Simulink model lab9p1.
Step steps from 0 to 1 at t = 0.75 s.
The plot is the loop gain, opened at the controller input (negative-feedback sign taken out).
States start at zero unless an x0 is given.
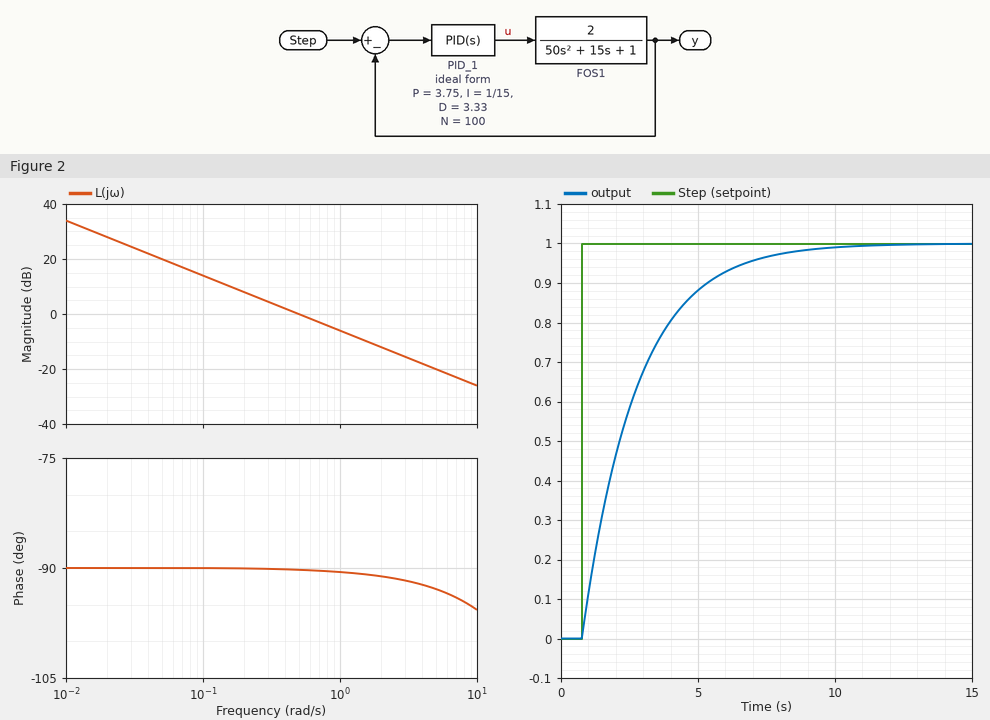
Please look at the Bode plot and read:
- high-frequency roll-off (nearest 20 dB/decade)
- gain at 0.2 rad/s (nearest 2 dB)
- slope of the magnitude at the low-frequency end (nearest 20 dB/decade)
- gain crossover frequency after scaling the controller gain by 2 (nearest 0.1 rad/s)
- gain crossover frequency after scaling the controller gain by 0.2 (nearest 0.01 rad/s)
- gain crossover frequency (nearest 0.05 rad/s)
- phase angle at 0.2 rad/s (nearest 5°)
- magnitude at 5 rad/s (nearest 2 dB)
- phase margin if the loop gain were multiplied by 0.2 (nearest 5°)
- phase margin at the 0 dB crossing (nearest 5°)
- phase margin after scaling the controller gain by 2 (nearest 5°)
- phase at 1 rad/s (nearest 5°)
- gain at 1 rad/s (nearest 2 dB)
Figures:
-20 dB/decade
8 dB
-20 dB/decade
1.0 rad/s
0.10 rad/s
0.50 rad/s
-90°
-20 dB
90°
90°
90°
-90°
-6 dB
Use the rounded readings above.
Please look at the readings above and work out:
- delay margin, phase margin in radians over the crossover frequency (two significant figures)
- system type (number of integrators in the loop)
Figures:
3.1 s
1
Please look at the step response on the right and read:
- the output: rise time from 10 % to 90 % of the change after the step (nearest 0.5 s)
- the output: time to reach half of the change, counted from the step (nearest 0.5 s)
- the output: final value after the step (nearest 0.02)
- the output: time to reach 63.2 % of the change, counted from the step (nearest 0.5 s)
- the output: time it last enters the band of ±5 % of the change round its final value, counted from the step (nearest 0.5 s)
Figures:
4.5 s
1.5 s
1.00
2.0 s
6.0 s
